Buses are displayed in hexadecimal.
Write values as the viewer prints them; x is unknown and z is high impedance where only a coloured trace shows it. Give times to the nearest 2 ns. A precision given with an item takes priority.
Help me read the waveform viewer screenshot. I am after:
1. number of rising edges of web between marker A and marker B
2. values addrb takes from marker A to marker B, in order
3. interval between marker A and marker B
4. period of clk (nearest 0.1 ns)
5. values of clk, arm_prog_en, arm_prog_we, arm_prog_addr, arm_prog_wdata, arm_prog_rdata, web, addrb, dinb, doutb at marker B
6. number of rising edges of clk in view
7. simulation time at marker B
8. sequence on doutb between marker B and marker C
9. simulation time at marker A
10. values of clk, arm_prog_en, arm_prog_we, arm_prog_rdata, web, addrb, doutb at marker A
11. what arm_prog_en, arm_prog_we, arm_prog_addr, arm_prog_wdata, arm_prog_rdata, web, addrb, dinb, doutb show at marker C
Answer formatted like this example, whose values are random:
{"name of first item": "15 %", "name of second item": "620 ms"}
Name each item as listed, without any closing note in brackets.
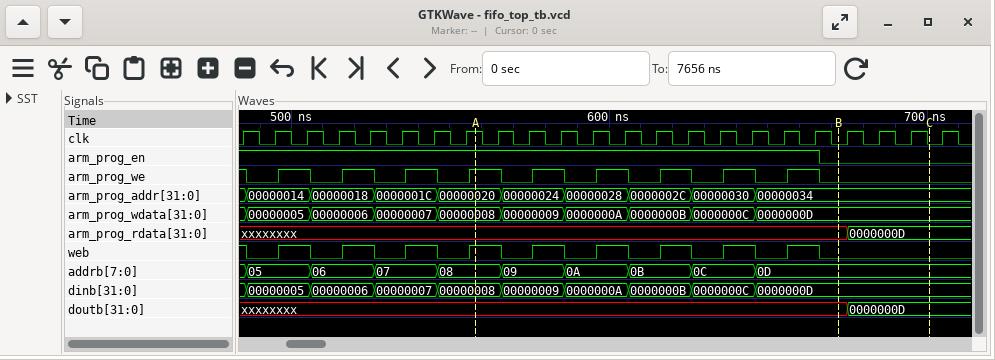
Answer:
{"number of rising edges of web between marker A and marker B": "5", "values addrb takes from marker A to marker B, in order": "08, 09, 0A, 0B, 0C, 0D", "interval between marker A and marker B": "114 ns", "period of clk": "10 ns", "values of clk, arm_prog_en, arm_prog_we, arm_prog_addr, arm_prog_wdata, arm_prog_rdata, web, addrb, dinb, doutb at marker B": "clk=0, arm_prog_en=0, arm_prog_we=0, arm_prog_addr=00000034, arm_prog_wdata=0000000D, arm_prog_rdata=xxxxxxxx, web=0, addrb=0D, dinb=0000000D, doutb=xxxxxxxx", "number of rising edges of clk in view": "23", "simulation time at marker B": "672 ns", "sequence on doutb between marker B and marker C": "xxxxxxxx, 0000000D", "simulation time at marker A": "558 ns", "values of clk, arm_prog_en, arm_prog_we, arm_prog_rdata, web, addrb, doutb at marker A": "clk=1, arm_prog_en=1, arm_prog_we=1, arm_prog_rdata=xxxxxxxx, web=1, addrb=08, doutb=xxxxxxxx", "what arm_prog_en, arm_prog_we, arm_prog_addr, arm_prog_wdata, arm_prog_rdata, web, addrb, dinb, doutb show at marker C": "arm_prog_en=0, arm_prog_we=0, arm_prog_addr=00000034, arm_prog_wdata=0000000D, arm_prog_rdata=0000000D, web=0, addrb=0D, dinb=0000000D, doutb=0000000D"}
